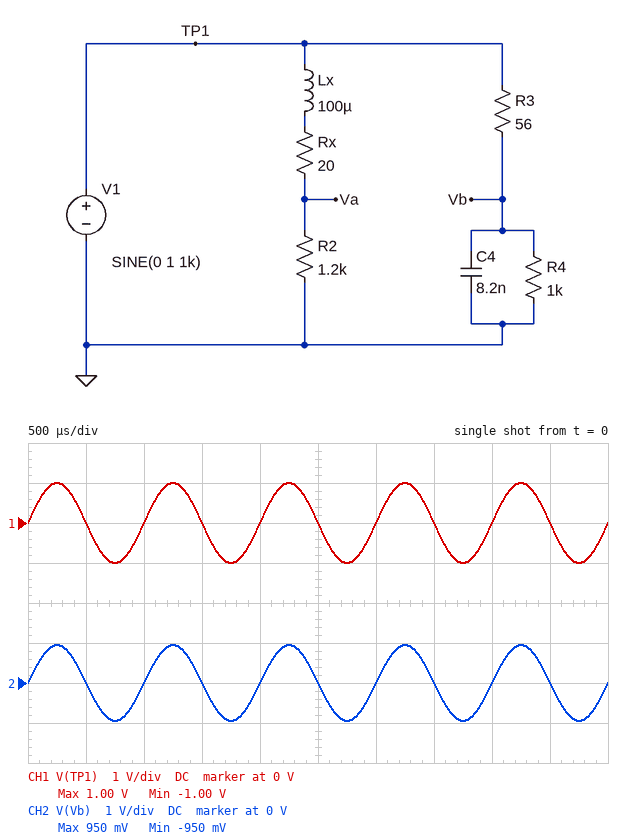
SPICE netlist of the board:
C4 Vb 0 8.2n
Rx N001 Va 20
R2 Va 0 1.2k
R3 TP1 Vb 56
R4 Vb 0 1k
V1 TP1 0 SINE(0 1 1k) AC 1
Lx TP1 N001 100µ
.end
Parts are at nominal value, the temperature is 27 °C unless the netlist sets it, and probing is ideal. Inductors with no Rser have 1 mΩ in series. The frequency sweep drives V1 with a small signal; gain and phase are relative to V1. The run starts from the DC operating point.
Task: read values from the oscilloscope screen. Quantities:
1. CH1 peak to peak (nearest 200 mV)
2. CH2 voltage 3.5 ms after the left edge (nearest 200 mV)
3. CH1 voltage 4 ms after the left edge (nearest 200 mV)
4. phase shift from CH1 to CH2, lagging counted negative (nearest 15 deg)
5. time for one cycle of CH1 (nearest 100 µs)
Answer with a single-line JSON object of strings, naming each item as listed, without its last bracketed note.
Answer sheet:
{"CH1 peak to peak": "2.0 V", "CH2 voltage 3.5 ms after the left edge": "0 V", "CH1 voltage 4 ms after the left edge": "0 V", "phase shift from CH1 to CH2, lagging counted negative": "0 deg", "time for one cycle of CH1": "1.0 ms"}
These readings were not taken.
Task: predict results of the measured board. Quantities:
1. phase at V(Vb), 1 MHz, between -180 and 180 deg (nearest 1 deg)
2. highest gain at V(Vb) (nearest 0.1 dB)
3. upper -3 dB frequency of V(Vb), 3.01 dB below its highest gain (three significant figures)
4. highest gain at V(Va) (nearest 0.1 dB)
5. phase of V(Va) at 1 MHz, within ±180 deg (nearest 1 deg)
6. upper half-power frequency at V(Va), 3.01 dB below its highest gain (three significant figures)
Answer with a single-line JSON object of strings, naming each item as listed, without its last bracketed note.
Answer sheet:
{"phase at V(Vb), 1 MHz, between -180 and 180 deg": "-70 deg", "highest gain at V(Vb)": "-0.5 dB", "upper -3 dB frequency of V(Vb), 3.01 dB below its highest gain": "366 kHz", "highest gain at V(Va)": "-0.1 dB", "phase of V(Va) at 1 MHz, within ±180 deg": "-27 deg", "upper half-power frequency at V(Va), 3.01 dB below its highest gain": "1.94 MHz"}
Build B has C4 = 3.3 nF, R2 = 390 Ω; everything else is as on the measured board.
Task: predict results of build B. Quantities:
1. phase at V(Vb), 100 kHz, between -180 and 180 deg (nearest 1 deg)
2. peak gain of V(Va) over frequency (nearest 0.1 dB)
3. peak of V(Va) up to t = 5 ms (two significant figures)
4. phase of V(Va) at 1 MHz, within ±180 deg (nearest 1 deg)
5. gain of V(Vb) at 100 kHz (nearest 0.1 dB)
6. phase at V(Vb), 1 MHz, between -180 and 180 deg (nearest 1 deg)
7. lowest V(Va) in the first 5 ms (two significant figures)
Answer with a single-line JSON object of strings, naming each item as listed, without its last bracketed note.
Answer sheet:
{"phase at V(Vb), 100 kHz, between -180 and 180 deg": "-6 deg", "peak gain of V(Va) over frequency": "-0.4 dB", "peak of V(Va) up to t = 5 ms": "950 mV", "phase of V(Va) at 1 MHz, within ±180 deg": "-57 deg", "gain of V(Vb) at 100 kHz": "-0.5 dB", "phase at V(Vb), 1 MHz, between -180 and 180 deg": "-48 deg", "lowest V(Va) in the first 5 ms": "-950 mV"}
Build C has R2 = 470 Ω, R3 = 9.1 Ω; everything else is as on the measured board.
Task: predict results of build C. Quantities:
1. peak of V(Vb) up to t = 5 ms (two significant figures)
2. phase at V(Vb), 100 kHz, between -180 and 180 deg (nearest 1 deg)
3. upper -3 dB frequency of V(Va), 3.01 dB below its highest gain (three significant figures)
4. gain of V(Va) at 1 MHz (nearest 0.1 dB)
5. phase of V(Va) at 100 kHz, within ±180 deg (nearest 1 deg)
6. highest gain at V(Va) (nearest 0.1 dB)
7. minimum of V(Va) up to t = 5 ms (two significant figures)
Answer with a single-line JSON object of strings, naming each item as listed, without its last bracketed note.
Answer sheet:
{"peak of V(Vb) up to t = 5 ms": "990 mV", "phase at V(Vb), 100 kHz, between -180 and 180 deg": "-3 deg", "upper -3 dB frequency of V(Va), 3.01 dB below its highest gain": "780 kHz", "gain of V(Va) at 1 MHz": "-4.6 dB", "phase of V(Va) at 100 kHz, within ±180 deg": "-7 deg", "highest gain at V(Va)": "-0.4 dB", "minimum of V(Va) up to t = 5 ms": "-960 mV"}
